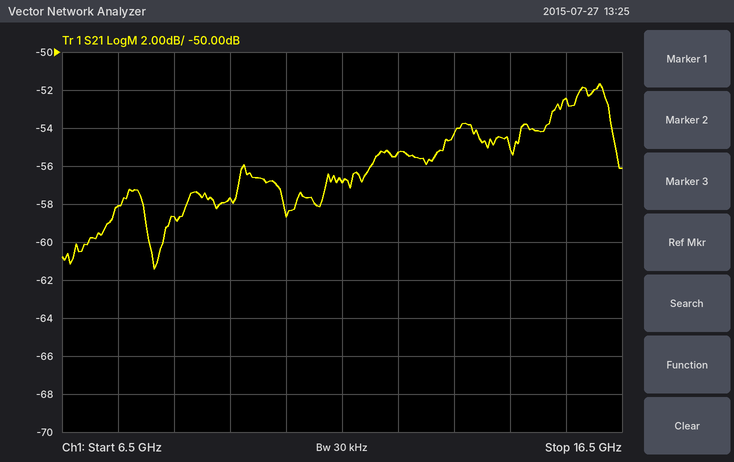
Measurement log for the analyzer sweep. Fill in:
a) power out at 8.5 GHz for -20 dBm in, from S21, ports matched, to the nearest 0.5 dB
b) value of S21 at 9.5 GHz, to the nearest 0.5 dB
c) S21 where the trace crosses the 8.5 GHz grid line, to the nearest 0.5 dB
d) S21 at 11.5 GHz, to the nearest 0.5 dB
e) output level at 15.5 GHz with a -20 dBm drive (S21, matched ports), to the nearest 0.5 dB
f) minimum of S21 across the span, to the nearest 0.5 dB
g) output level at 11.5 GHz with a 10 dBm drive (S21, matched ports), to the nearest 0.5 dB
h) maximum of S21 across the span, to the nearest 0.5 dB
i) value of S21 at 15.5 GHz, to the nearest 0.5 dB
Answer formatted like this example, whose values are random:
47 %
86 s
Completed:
-78.5 dBm
-57.5 dB
-58.5 dB
-57.0 dB
-72.5 dBm
-61.5 dB
-47.0 dBm
-51.5 dB
-52.5 dB
